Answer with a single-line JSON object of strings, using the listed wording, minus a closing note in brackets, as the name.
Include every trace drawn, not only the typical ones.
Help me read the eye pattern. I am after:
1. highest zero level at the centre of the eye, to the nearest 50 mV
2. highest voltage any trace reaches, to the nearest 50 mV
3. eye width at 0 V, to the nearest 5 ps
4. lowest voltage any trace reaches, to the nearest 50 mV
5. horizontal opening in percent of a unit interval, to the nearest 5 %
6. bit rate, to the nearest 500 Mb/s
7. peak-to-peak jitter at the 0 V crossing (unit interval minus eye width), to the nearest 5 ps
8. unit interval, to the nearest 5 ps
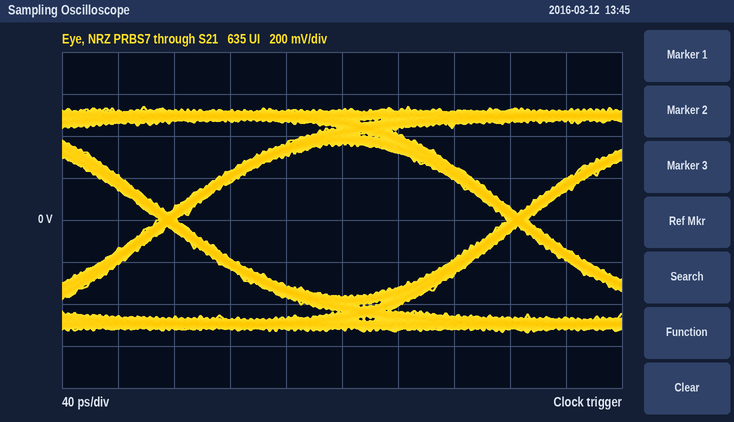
{"highest zero level at the centre of the eye, to the nearest 50 mV": "-350 mV", "highest voltage any trace reaches, to the nearest 50 mV": "550 mV", "eye width at 0 V, to the nearest 5 ps": "235 ps", "lowest voltage any trace reaches, to the nearest 50 mV": "-550 mV", "horizontal opening in percent of a unit interval, to the nearest 5 %": "95 %", "bit rate, to the nearest 500 Mb/s": "4.0 Gb/s", "peak-to-peak jitter at the 0 V crossing (unit interval minus eye width), to the nearest 5 ps": "15 ps", "unit interval, to the nearest 5 ps": "250 ps"}
